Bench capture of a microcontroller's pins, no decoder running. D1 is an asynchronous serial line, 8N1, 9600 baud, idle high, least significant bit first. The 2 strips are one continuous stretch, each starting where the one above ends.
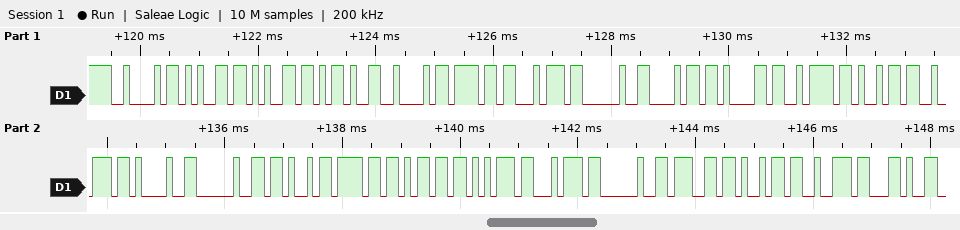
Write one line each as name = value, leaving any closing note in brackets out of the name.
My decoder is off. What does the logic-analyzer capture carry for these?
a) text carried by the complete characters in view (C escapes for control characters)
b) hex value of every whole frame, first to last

text carried by the complete characters in view = "Bee-Bot hazir! Komut gir,"
hex value of every whole frame, first to last = 42 65 65 2D 42 6F 74 20 68 61 7A 69 72 21 20 4B 6F 6D 75 74 20 67 69 72 2C
